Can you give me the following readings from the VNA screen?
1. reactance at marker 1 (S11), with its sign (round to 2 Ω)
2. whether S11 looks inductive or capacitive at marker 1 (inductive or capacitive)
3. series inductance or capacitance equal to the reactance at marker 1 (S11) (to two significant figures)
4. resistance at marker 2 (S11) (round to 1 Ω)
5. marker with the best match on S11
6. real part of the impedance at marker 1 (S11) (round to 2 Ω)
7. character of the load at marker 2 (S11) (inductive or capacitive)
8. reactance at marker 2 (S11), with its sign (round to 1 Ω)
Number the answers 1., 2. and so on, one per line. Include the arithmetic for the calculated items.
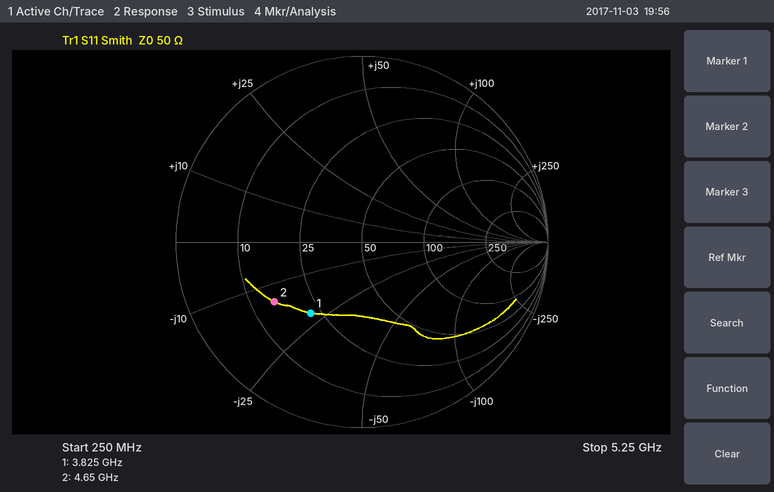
1. -22 Ω
2. capacitive
3. C = 1/(2π × 3.825 GHz × 22 Ω) ≈ 1.9 pF
4. 15 Ω
5. marker 1
6. 22 Ω
7. capacitive
8. -14 Ω
